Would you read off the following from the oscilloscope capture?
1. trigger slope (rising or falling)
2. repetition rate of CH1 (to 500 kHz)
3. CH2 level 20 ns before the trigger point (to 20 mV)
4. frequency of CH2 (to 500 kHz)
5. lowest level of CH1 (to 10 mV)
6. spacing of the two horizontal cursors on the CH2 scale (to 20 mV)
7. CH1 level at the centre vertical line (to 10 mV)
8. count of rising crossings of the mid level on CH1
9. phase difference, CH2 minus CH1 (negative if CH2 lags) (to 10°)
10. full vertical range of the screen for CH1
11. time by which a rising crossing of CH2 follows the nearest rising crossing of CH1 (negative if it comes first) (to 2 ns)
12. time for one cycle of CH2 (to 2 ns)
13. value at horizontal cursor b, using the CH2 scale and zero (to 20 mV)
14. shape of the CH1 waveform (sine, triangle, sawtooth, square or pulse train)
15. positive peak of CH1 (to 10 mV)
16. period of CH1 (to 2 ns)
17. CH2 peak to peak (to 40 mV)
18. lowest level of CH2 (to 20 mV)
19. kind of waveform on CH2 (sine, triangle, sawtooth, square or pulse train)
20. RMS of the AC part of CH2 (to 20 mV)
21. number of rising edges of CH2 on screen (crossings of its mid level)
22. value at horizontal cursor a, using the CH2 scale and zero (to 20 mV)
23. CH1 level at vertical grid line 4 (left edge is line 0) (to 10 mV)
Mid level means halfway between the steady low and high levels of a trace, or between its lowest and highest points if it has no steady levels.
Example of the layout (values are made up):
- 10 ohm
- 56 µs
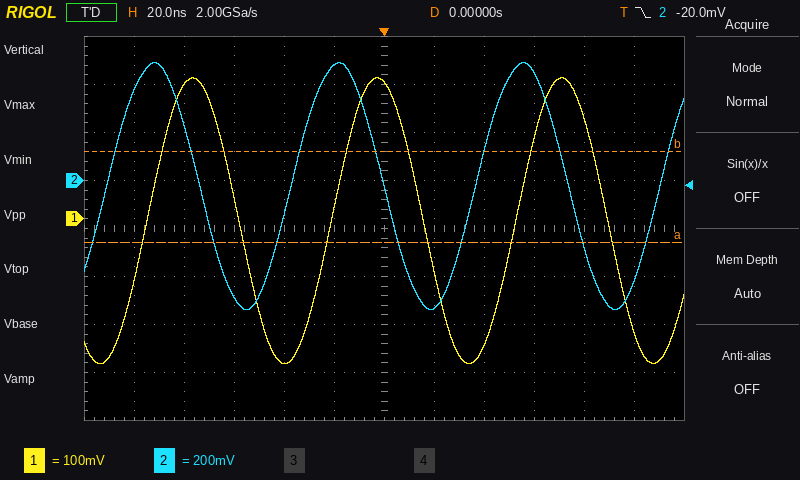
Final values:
- falling
- 13.5 MHz
- 480 mV
- 13.5 MHz
- -300 mV
- 380 mV
- 280 mV
- 3
- +80°
- 800 mV
- -16 ns
- 74 ns
- 120 mV
- sine
- 290 mV
- 74 ns
- 1.04 V
- -540 mV
- sine
- 360 mV
- 4
- -260 mV
- -300 mV
